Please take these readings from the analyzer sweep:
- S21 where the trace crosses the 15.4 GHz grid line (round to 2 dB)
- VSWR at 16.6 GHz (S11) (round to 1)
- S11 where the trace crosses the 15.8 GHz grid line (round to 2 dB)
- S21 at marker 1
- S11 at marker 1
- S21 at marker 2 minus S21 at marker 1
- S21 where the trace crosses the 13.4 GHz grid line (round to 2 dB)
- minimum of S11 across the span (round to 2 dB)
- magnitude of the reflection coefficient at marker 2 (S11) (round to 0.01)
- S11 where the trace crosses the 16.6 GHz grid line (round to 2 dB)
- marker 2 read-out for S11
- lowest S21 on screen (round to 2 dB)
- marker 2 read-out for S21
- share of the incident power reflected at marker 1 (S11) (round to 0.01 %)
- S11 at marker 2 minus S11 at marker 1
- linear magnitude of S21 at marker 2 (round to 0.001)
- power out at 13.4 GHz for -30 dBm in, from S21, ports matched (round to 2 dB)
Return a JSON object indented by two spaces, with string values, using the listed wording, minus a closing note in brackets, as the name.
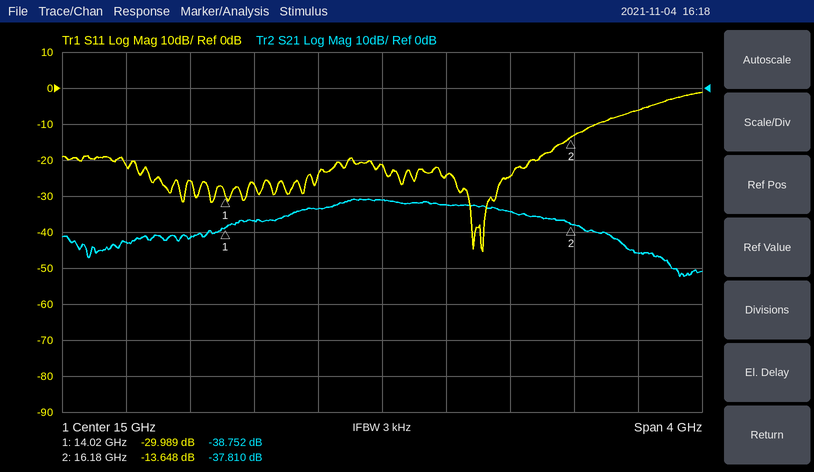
{
  "S21 where the trace crosses the 15.4 GHz grid line": "-32 dB",
  "VSWR at 16.6 GHz (S11)": "3",
  "S11 where the trace crosses the 15.8 GHz grid line": "-24 dB",
  "S21 at marker 1": "-38.752 dB",
  "S11 at marker 1": "-29.989 dB",
  "S21 at marker 2 minus S21 at marker 1": "0.942 dB",
  "S21 where the trace crosses the 13.4 GHz grid line": "-42 dB",
  "minimum of S11 across the span": "-46 dB",
  "magnitude of the reflection coefficient at marker 2 (S11)": "0.21",
  "S11 where the trace crosses the 16.6 GHz grid line": "-6 dB",
  "marker 2 read-out for S11": "-13.648 dB",
  "lowest S21 on screen": "-52 dB",
  "marker 2 read-out for S21": "-37.810 dB",
  "share of the incident power reflected at marker 1 (S11)": "0.10 %",
  "S11 at marker 2 minus S11 at marker 1": "16.341 dB",
  "linear magnitude of S21 at marker 2": "0.013",
  "power out at 13.4 GHz for -30 dBm in, from S21, ports matched": "-72 dBm"
}
